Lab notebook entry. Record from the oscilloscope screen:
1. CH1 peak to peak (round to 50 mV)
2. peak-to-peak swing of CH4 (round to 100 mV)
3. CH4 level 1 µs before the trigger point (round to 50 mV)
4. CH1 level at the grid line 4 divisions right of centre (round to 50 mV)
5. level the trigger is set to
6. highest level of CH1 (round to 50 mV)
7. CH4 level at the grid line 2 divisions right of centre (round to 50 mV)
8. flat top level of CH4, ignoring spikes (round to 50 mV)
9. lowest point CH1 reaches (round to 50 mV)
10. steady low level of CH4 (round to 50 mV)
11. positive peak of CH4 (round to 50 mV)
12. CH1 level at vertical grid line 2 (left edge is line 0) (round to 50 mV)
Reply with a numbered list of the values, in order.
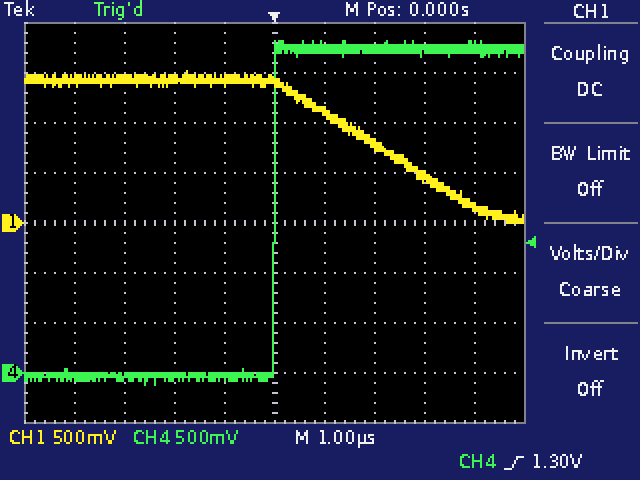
1. 1.50 V
2. 3.40 V
3. -50 mV
4. 150 mV
5. 1.30 V
6. 1.50 V
7. 3.25 V
8. 3.25 V
9. 0 mV
10. -50 mV
11. 3.30 V
12. 1.45 V
